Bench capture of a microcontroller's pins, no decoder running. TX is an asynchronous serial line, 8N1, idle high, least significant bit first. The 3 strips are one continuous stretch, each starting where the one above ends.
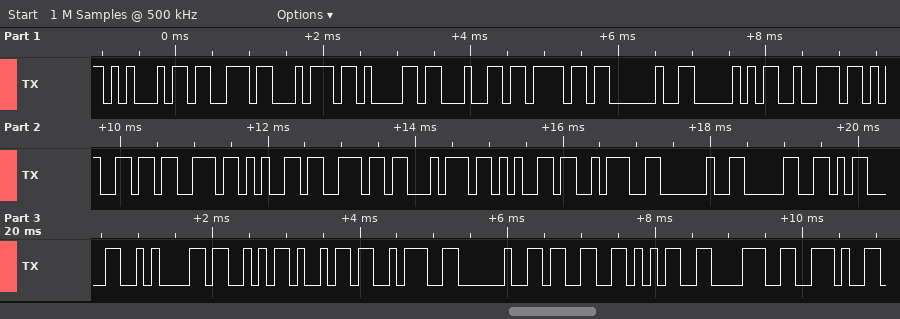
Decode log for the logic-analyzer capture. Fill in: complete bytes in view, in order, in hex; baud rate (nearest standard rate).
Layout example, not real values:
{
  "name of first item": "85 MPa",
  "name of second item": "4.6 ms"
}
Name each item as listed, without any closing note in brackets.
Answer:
{
  "complete bytes in view, in order, in hex": "0x45 0x73 0x74 0x61 0x64 0x6F 0x20 0x50 0x72 0x65 0x73 0x65 0x6E 0x74 0x65 0x3A 0x20 0x30 0x0D 0x0A 0x53 0x69 0x3A 0x20 0x33 0x35 0x38 0x2E",
  "baud rate": "9600 baud"
}
